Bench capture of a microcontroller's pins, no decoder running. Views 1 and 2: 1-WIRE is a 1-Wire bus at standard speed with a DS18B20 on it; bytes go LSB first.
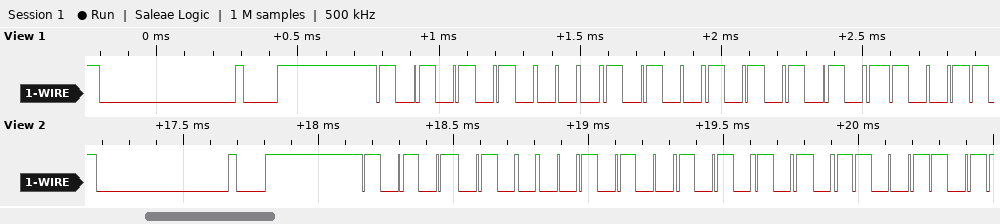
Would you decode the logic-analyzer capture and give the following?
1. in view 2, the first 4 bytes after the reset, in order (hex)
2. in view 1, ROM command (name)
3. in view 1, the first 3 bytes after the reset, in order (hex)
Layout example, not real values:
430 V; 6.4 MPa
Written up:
55 28 55 B3; Match ROM; 55 28 55
